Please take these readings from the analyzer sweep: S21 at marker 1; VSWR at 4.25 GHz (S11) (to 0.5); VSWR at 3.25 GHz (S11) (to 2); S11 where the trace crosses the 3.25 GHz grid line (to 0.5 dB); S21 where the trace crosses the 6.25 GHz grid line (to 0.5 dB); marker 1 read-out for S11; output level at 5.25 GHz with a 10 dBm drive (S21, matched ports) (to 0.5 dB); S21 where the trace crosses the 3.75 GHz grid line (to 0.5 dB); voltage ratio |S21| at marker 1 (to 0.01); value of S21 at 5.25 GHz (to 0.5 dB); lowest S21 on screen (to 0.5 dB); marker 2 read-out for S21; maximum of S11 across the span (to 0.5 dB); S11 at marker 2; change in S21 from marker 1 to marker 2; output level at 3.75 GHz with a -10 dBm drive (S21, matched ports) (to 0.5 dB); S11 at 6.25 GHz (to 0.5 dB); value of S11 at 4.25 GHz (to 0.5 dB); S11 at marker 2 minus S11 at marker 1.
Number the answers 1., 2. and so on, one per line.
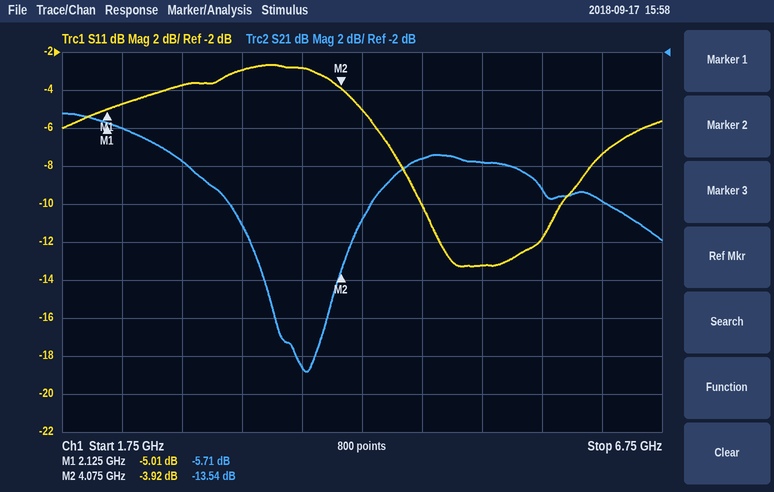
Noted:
1. -5.71 dB
2. 3.5
3. 6
4. -3.0 dB
5. -10.0 dB
6. -5.01 dB
7. 2.0 dBm
8. -18.5 dB
9. 0.52
10. -8.0 dB
11. -19.0 dB
12. -13.54 dB
13. -2.5 dB
14. -3.92 dB
15. -7.83 dB
16. -28.5 dBm
17. -7.5 dB
18. -5.0 dB
19. 1.09 dB
